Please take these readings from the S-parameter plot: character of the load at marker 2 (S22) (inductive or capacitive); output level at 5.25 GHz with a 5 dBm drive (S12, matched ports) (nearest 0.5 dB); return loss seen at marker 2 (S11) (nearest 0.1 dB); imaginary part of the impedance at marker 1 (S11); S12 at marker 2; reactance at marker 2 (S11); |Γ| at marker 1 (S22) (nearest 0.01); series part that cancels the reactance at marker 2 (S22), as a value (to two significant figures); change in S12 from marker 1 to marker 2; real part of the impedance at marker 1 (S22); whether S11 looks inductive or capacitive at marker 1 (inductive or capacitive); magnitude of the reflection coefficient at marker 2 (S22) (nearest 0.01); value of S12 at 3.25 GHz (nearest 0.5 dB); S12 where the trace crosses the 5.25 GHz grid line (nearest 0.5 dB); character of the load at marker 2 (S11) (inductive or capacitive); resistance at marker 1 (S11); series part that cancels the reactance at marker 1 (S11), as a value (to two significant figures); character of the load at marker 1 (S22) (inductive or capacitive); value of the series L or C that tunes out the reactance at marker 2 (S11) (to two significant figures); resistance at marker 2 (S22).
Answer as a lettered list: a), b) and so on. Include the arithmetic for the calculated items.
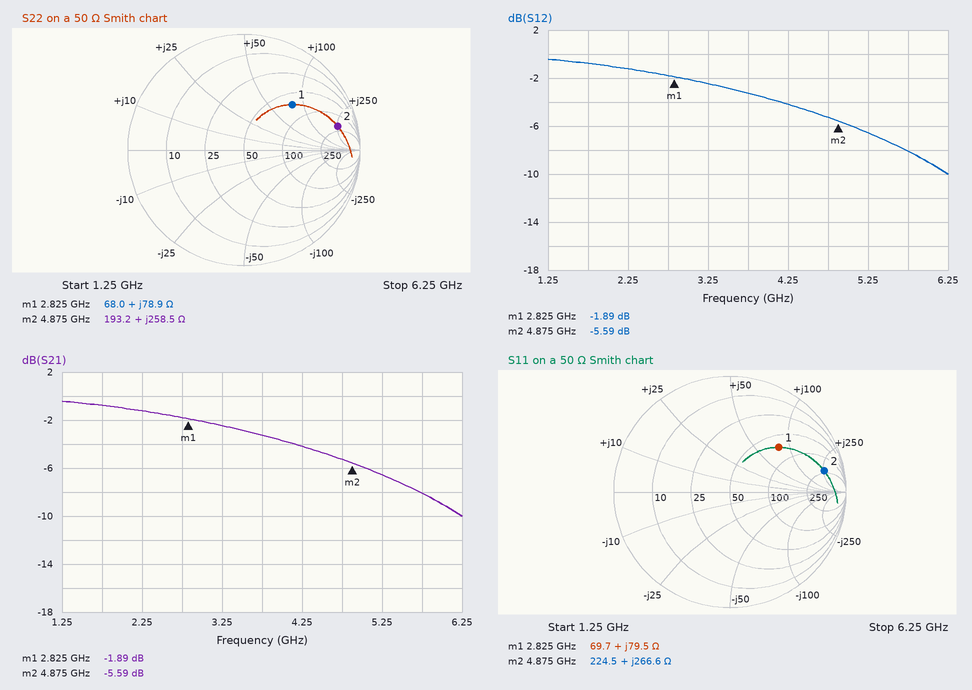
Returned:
a) inductive
b) 5 dBm + (-6.5 dB) = -1.5 dBm
c) 1.6 dB
d) +79.5 Ω
e) -5.59 dB
f) +266.6 Ω
g) 0.57
h) C = 1/(2π × 4.875 GHz × 258.5 Ω) ≈ 126 fF, so 130 fF to two significant figures
i) -5.59 − (-1.89) = -3.70 dB
j) 68.0 Ω
k) inductive
l) 0.83
m) -2.5 dB
n) -6.5 dB
o) inductive
p) 69.7 Ω
q) C = 1/(2π × 2.825 GHz × 79.5 Ω) ≈ 709 fF, so 710 fF to two significant figures
r) inductive
s) C = 1/(2π × 4.875 GHz × 266.6 Ω) ≈ 122 fF, so 120 fF to two significant figures
t) 193.2 Ω
